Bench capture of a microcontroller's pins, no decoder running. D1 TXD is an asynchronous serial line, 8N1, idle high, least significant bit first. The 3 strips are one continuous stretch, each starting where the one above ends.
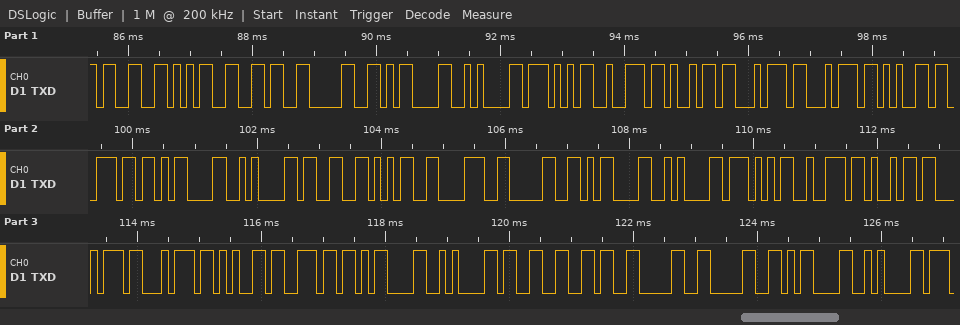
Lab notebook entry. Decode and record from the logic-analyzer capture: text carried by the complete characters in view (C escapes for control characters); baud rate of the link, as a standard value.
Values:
"3560\r\nWritten\r\n3580\r\nWritten\r\n3600\r\n"
9600 baud
